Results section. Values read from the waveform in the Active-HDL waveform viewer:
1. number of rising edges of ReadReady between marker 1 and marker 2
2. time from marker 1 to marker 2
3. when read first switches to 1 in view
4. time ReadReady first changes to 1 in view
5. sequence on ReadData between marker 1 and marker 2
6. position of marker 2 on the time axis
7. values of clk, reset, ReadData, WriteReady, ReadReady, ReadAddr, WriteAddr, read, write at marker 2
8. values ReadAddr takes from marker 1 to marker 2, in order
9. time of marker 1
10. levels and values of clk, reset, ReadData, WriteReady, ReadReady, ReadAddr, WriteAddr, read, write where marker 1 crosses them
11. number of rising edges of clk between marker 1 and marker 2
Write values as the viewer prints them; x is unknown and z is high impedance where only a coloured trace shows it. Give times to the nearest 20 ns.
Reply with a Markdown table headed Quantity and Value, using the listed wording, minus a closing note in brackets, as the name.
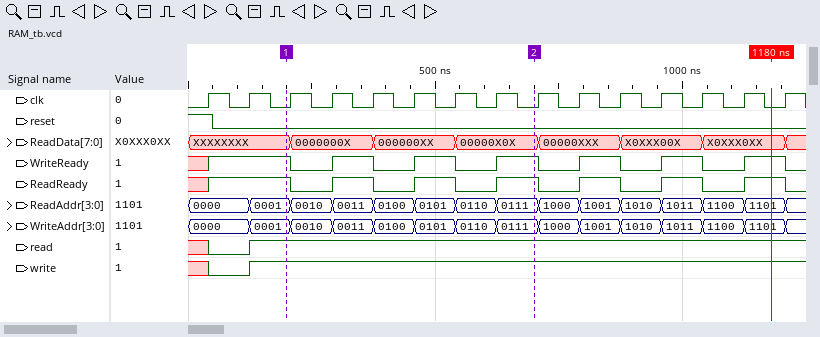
| Quantity | Value |
|---|---|
| number of rising edges of ReadReady between marker 1 and marker 2 | 3 |
| time from marker 1 to marker 2 | 500 ns |
| when read first switches to 1 in view | 120 ns |
| time ReadReady first changes to 1 in view | 40 ns |
| sequence on ReadData between marker 1 and marker 2 | XXXXXXXX, 0000000X, 000000XX, 00000X0X |
| position of marker 2 on the time axis | 700 ns |
| values of clk, reset, ReadData, WriteReady, ReadReady, ReadAddr, WriteAddr, read, write at marker 2 | clk=0, reset=0, ReadData=00000X0X, WriteReady=1, ReadReady=1, ReadAddr=0111, WriteAddr=0111, read=1, write=1 |
| values ReadAddr takes from marker 1 to marker 2, in order | 0001, 0010, 0011, 0100, 0101, 0110, 0111 |
| time of marker 1 | 200 ns |
| levels and values of clk, reset, ReadData, WriteReady, ReadReady, ReadAddr, WriteAddr, read, write where marker 1 crosses them | clk=0, reset=0, ReadData=XXXXXXXX, WriteReady=1, ReadReady=1, ReadAddr=0001, WriteAddr=0001, read=1, write=1 |
| number of rising edges of clk between marker 1 and marker 2 | 6 |
